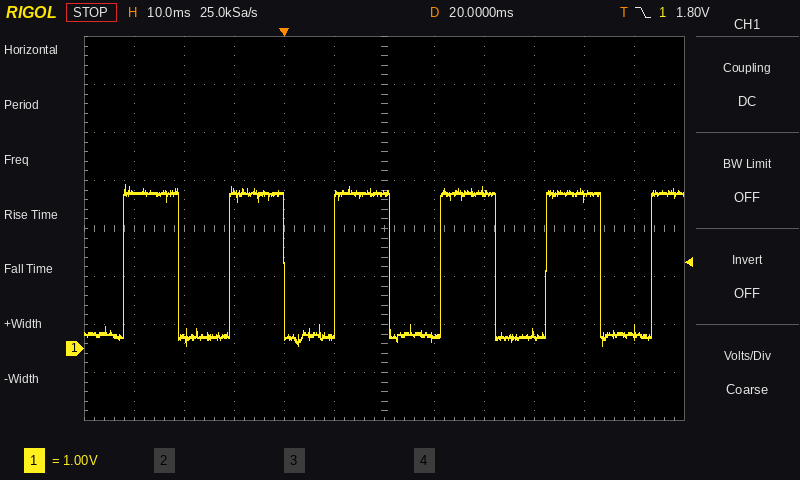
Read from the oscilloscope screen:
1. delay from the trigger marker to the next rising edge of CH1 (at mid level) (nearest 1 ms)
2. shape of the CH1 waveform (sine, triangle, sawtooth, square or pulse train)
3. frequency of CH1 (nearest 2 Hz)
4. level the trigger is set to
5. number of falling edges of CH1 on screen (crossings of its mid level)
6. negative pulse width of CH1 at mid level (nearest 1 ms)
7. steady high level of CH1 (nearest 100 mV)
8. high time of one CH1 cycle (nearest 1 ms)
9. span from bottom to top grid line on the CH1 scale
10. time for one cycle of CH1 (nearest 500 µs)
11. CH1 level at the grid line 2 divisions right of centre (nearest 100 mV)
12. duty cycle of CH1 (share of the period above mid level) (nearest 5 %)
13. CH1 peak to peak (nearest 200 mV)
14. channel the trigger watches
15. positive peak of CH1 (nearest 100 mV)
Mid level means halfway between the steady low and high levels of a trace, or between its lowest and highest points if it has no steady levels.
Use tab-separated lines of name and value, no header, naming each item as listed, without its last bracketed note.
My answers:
delay from the trigger marker to the next rising edge of CH1 (at mid level)	10 ms
shape of the CH1 waveform	square
frequency of CH1	48 Hz
level the trigger is set to	1.80 V
number of falling edges of CH1 on screen	5
negative pulse width of CH1 at mid level	10 ms
steady high level of CH1	3.2 V
high time of one CH1 cycle	11 ms
span from bottom to top grid line on the CH1 scale	8 V
time for one cycle of CH1	21.0 ms
CH1 level at the grid line 2 divisions right of centre	3.3 V
duty cycle of CH1 (share of the period above mid level)	50 %
CH1 peak to peak	3.4 V
channel the trigger watches	CH1
positive peak of CH1	3.4 V
